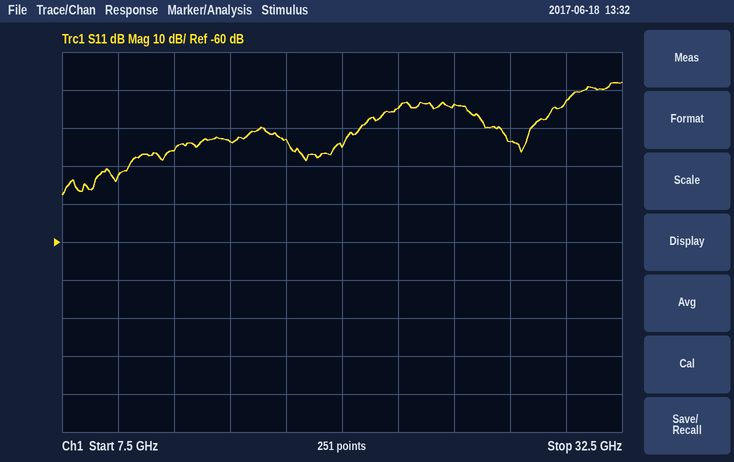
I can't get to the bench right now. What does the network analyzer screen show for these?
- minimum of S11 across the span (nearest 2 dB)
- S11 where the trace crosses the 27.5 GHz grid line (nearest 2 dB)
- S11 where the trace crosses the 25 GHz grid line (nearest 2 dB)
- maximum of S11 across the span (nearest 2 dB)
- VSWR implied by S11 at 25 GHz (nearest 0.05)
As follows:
-48 dB
-34 dB
-24 dB
-18 dB
1.15
